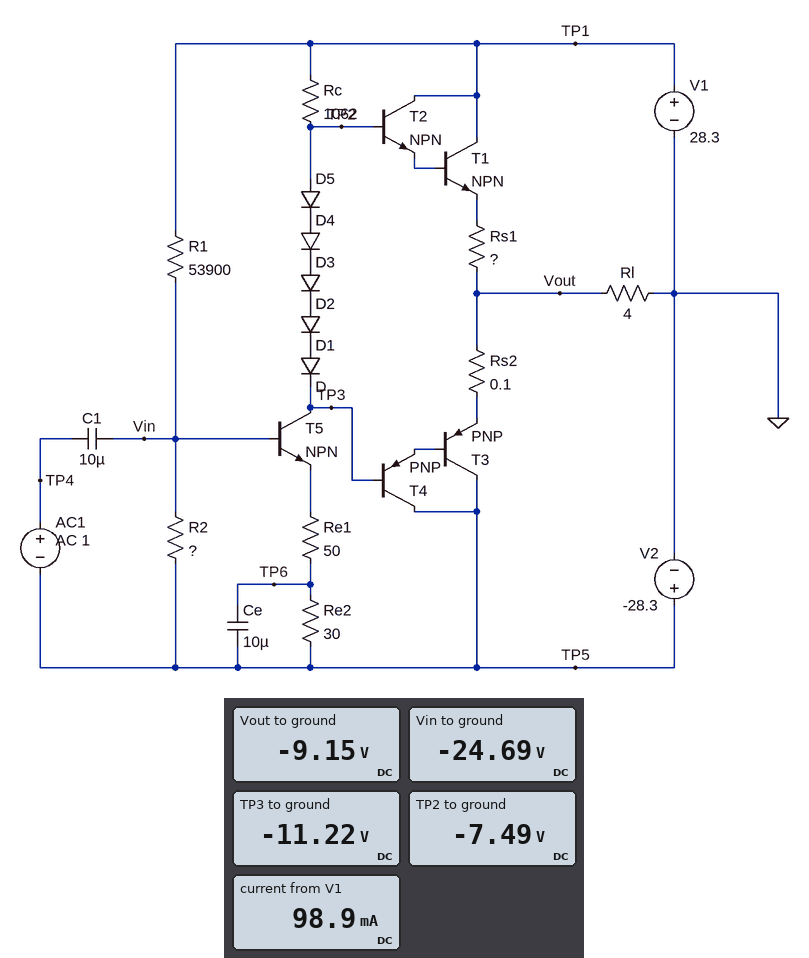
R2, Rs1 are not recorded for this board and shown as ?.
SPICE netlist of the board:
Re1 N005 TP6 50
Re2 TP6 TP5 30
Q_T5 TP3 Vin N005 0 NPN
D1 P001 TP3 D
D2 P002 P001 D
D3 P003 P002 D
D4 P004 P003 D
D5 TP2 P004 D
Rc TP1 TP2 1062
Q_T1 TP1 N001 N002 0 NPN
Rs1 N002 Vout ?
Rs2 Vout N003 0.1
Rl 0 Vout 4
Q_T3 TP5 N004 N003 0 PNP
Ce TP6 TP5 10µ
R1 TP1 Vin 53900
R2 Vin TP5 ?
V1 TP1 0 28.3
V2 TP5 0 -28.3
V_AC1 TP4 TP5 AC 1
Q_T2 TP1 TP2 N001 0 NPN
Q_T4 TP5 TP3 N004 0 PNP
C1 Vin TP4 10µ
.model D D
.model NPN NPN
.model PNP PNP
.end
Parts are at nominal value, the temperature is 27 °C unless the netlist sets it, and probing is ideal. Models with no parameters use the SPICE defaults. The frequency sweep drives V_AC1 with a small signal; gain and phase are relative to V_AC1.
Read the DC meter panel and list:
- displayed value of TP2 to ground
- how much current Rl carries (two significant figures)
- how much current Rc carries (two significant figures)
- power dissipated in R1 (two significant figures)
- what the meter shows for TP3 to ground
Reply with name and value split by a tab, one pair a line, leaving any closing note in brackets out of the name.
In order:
displayed value of TP2 to ground	-7.49 V
how much current Rl carries	2.3 A
how much current Rc carries	34 mA
power dissipated in R1	52 mW
what the meter shows for TP3 to ground	-11.22 V
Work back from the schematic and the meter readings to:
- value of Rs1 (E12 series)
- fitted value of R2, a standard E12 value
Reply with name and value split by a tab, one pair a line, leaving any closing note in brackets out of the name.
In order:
value of Rs1	0.33 Ω
fitted value of R2, a standard E12 value	5.6 kΩ
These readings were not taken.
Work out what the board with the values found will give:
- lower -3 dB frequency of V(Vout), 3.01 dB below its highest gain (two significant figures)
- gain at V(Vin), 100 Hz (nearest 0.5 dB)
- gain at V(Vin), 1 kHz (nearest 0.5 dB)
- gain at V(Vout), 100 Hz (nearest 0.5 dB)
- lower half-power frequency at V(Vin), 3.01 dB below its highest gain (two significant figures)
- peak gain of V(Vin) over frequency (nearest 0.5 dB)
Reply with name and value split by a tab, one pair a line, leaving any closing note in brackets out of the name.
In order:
lower -3 dB frequency of V(Vout), 3.01 dB below its highest gain	390 Hz
gain at V(Vin), 100 Hz	0 dB
gain at V(Vin), 1 kHz	0 dB
gain at V(Vout), 100 Hz	22.0 dB
lower half-power frequency at V(Vin), 3.01 dB below its highest gain	5.1 Hz
peak gain of V(Vin) over frequency	0 dB
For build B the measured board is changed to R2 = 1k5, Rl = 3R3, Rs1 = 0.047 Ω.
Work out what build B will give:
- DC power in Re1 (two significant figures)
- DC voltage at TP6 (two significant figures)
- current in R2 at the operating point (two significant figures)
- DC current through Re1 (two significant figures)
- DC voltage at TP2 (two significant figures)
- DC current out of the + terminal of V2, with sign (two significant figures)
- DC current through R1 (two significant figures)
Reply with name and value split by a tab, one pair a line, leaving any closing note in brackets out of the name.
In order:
DC power in Re1	2.8 mW
DC voltage at TP6	-28 V
current in R2 at the operating point	950 µA
DC current through Re1	7.5 mA
DC voltage at TP2	20 V
DC current out of the + terminal of V2, with sign	-9.1 mA
DC current through R1	1.0 mA
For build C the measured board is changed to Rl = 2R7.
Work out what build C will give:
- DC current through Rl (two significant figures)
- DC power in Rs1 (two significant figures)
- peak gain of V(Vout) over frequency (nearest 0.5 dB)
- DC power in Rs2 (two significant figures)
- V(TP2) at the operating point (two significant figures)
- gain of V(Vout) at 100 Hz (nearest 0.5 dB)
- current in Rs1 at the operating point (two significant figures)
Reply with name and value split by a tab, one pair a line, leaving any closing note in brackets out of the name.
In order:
DC current through Rl	3.3 A
DC power in Rs1	32 µW
peak gain of V(Vout) over frequency	25.5 dB
DC power in Rs2	1.1 W
V(TP2) at the operating point	-7.4 V
gain of V(Vout) at 100 Hz	21.5 dB
current in Rs1 at the operating point	9.9 mA
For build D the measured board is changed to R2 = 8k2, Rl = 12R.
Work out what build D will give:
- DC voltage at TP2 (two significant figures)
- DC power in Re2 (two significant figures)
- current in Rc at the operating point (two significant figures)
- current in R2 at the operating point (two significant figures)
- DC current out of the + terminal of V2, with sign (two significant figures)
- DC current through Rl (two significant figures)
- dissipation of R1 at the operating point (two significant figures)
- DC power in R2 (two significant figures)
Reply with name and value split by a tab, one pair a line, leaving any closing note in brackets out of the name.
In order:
DC voltage at TP2	-18 V
DC power in Re2	58 mW
current in Rc at the operating point	43 mA
current in R2 at the operating point	530 µA
DC current out of the + terminal of V2, with sign	-1.9 A
DC current through Rl	1.6 A
dissipation of R1 at the operating point	51 mW
DC power in R2	2.3 mW
